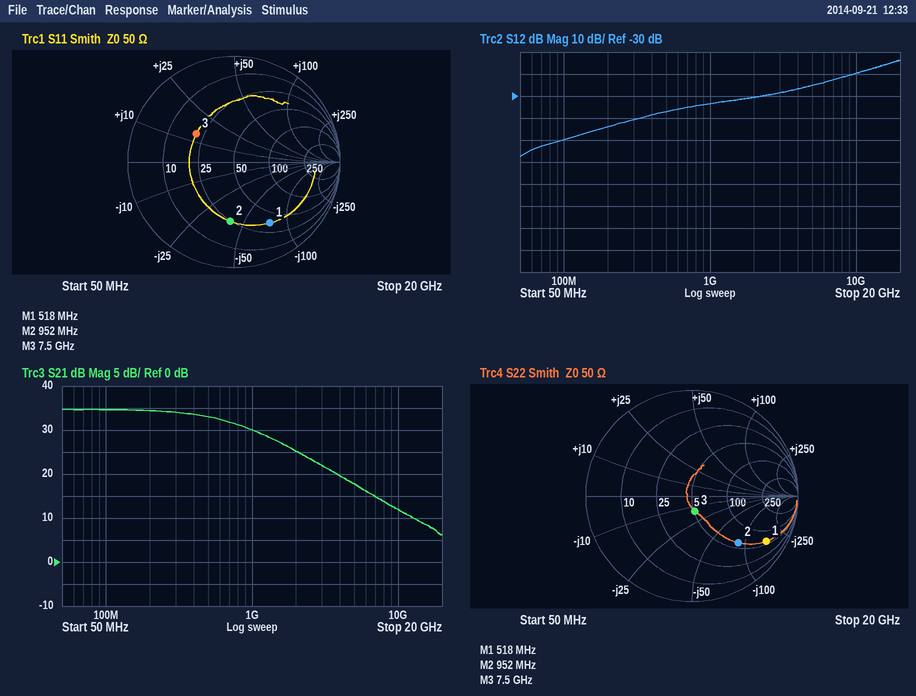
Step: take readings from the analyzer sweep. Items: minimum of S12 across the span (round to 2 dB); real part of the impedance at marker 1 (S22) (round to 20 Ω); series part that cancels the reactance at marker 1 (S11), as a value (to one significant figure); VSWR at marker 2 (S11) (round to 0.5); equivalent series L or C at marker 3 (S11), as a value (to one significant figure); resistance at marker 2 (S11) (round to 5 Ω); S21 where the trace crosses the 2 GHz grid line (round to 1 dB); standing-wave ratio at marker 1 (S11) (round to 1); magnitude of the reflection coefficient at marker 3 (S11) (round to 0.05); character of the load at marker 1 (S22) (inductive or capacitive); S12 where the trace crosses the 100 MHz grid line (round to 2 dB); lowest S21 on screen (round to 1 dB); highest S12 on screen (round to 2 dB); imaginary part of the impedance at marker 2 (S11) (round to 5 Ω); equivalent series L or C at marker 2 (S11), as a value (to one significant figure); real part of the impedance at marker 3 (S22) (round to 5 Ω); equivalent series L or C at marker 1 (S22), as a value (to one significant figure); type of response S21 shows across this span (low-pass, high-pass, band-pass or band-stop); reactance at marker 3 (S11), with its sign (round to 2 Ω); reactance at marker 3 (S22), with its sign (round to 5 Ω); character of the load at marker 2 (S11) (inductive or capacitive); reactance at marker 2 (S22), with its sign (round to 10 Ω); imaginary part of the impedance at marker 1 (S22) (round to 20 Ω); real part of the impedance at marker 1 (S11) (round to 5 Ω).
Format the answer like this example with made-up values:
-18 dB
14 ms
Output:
-58 dB
60 Ω
20 nH
3.5
300 pH
25 Ω
25 dB
5
0.45
capacitive
-50 dB
6 dB
-14 dB
-40 Ω
4 pF
50 Ω
2 pF
low-pass
+14 Ω
-15 Ω
capacitive
-90 Ω
-160 Ω
35 Ω
